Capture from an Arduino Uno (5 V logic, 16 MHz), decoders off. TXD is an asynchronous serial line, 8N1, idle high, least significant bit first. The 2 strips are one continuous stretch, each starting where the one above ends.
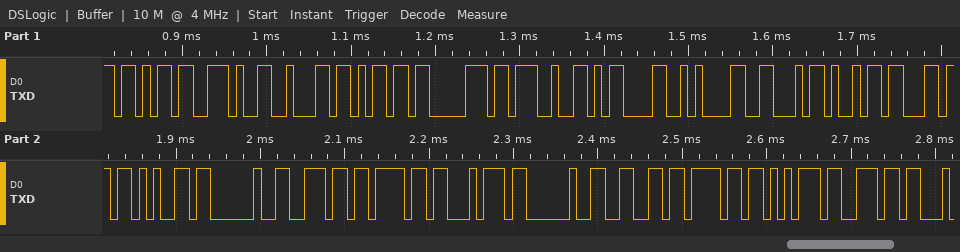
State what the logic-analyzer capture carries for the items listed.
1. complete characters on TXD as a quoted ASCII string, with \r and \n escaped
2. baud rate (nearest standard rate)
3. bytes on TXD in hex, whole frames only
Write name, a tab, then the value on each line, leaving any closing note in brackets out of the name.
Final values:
complete characters on TXD as a quoted ASCII string, with \r and \n escaped	"k.bmp'\r\nFile not foun"
baud rate	115200 baud
bytes on TXD in hex, whole frames only	6B 2E 62 6D 70 27 0D 0A 46 69 6C 65 20 6E 6F 74 20 66 6F 75 6E
